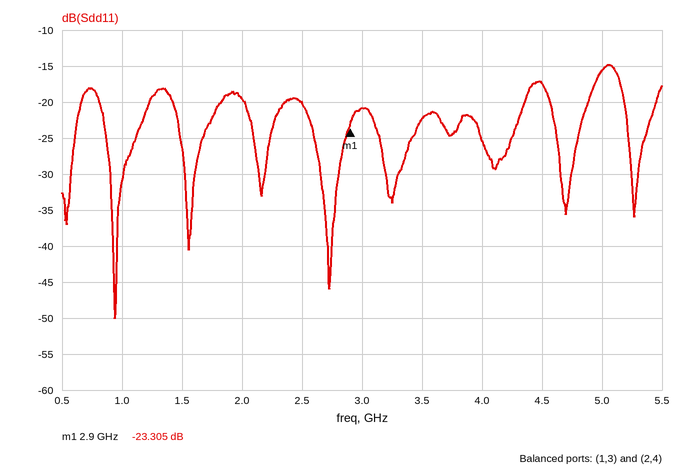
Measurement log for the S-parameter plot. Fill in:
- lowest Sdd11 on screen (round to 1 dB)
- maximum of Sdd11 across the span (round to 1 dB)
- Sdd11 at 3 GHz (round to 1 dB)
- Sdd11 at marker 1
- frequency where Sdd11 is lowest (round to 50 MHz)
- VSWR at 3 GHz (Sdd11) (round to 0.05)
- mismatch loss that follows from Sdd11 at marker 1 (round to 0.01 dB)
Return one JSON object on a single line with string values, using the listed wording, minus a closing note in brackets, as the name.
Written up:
{"lowest Sdd11 on screen": "-50 dB", "maximum of Sdd11 across the span": "-15 dB", "Sdd11 at 3 GHz": "-21 dB", "Sdd11 at marker 1": "-23.305 dB", "frequency where Sdd11 is lowest": "950 MHz", "VSWR at 3 GHz (Sdd11)": "1.20", "mismatch loss that follows from Sdd11 at marker 1": "0.02 dB"}
